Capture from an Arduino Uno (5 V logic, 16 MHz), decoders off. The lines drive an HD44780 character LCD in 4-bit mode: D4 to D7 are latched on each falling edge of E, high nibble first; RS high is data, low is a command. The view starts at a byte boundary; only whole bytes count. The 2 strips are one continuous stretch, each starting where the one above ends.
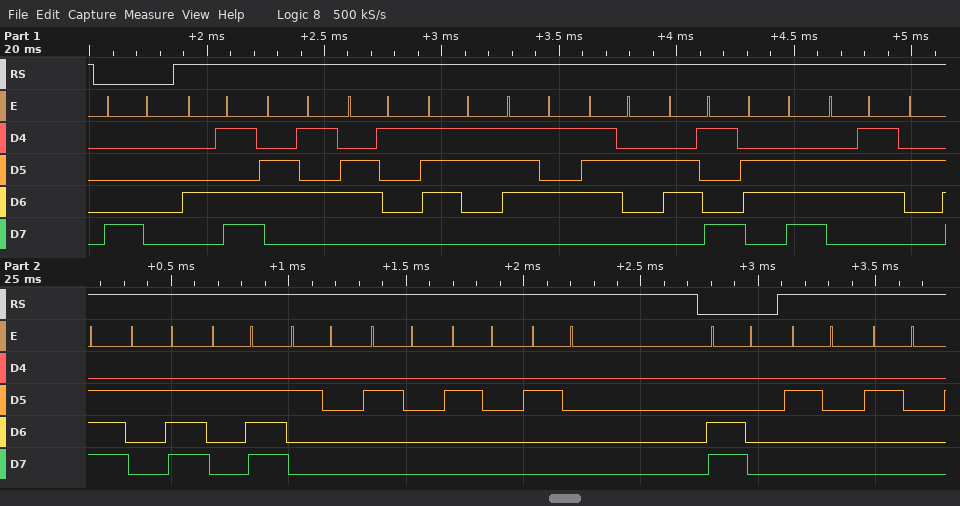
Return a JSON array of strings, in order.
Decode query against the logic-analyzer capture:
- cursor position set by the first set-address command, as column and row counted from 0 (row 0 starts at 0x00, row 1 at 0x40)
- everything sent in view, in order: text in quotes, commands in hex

["column 0, row 0", "0x80 \"Measuring...    \" 0xC0 \"  \""]
